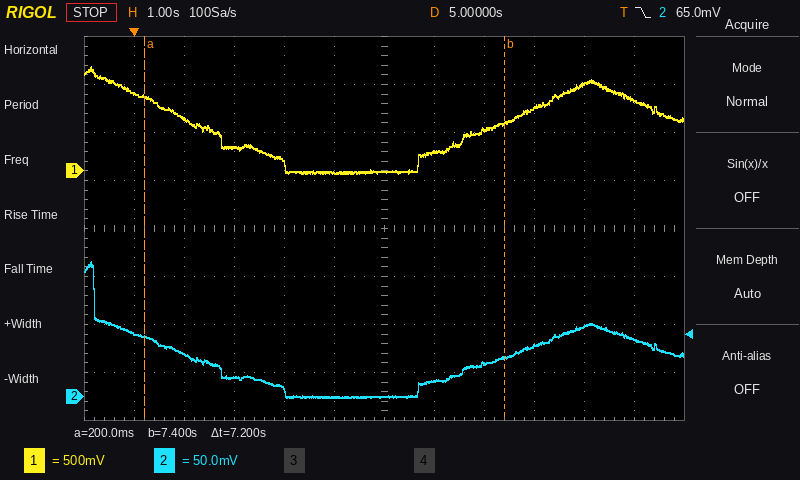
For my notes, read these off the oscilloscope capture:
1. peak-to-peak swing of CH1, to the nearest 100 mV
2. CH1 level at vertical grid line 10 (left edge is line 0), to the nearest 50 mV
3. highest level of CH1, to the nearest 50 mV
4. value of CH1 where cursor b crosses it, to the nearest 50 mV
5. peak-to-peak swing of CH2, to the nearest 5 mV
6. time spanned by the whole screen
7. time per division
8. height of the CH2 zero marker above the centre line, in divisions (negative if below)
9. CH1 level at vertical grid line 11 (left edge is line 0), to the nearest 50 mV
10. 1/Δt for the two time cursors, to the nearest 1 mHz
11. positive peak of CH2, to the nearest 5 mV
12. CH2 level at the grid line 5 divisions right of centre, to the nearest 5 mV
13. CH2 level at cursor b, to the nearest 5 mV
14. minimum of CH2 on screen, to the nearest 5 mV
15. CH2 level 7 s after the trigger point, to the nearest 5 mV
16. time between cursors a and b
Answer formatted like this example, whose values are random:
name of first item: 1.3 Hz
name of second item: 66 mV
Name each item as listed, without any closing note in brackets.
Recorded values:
peak-to-peak swing of CH1, to the nearest 100 mV: 1.10 V
CH1 level at vertical grid line 10 (left edge is line 0), to the nearest 50 mV: 900 mV
highest level of CH1, to the nearest 50 mV: 1.10 V
value of CH1 where cursor b crosses it, to the nearest 50 mV: 500 mV
peak-to-peak swing of CH2, to the nearest 5 mV: 140 mV
time spanned by the whole screen: 12 s
time per division: 1 s
height of the CH2 zero marker above the centre line, in divisions: -3.5 div
CH1 level at vertical grid line 11 (left edge is line 0), to the nearest 50 mV: 750 mV
1/Δt for the two time cursors, to the nearest 1 mHz: 139 mHz
positive peak of CH2, to the nearest 5 mV: 140 mV
CH2 level at the grid line 5 divisions right of centre, to the nearest 5 mV: 60 mV
CH2 level at cursor b, to the nearest 5 mV: 40 mV
minimum of CH2 on screen, to the nearest 5 mV: 0 mV
CH2 level 7 s after the trigger point, to the nearest 5 mV: 35 mV
time between cursors a and b: 7.2 s
